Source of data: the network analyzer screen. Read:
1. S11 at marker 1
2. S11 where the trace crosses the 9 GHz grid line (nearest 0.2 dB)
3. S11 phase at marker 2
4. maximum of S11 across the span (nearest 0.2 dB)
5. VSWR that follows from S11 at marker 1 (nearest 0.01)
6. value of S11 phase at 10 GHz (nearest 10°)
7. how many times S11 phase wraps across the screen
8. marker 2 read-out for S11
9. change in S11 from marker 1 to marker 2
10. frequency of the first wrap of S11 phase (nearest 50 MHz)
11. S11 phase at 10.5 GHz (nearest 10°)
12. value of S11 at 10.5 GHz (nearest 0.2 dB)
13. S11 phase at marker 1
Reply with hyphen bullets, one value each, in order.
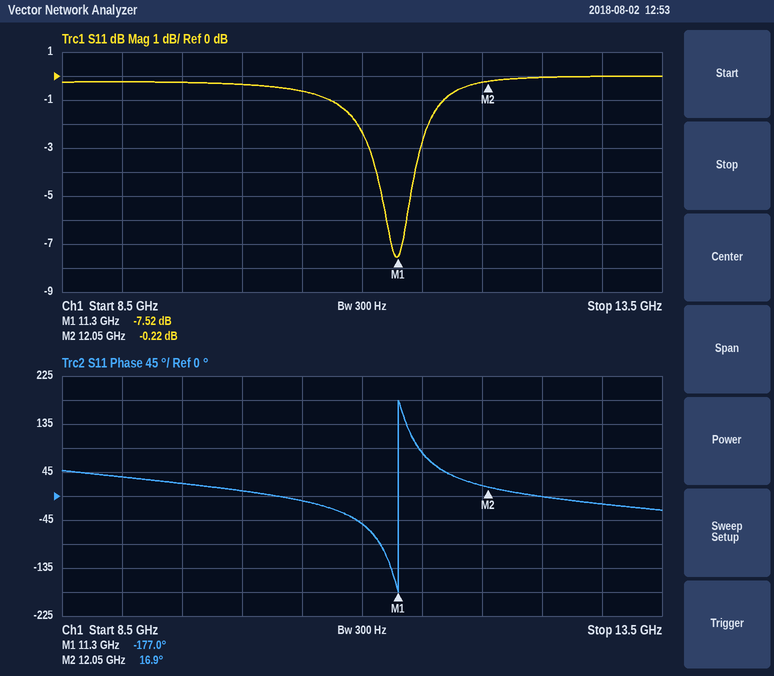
- -7.52 dB
- -0.2 dB
- 16.9°
- 0.0 dB
- 2.45
- 10°
- 1
- -0.22 dB
- 7.30 dB
- 11.30 GHz
- -10°
- -0.6 dB
- -177.0°
